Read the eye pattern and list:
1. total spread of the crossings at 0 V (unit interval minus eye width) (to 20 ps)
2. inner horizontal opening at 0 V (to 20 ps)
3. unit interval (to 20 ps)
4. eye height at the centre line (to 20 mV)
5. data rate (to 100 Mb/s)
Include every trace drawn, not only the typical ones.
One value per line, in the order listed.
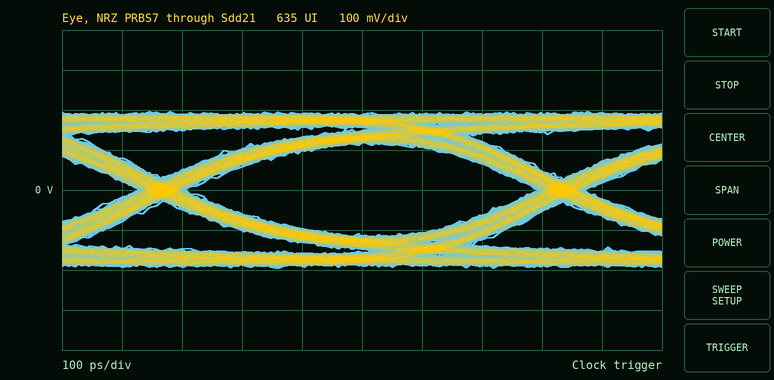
80 ps
580 ps
660 ps
240 mV
1.5 Gb/s
